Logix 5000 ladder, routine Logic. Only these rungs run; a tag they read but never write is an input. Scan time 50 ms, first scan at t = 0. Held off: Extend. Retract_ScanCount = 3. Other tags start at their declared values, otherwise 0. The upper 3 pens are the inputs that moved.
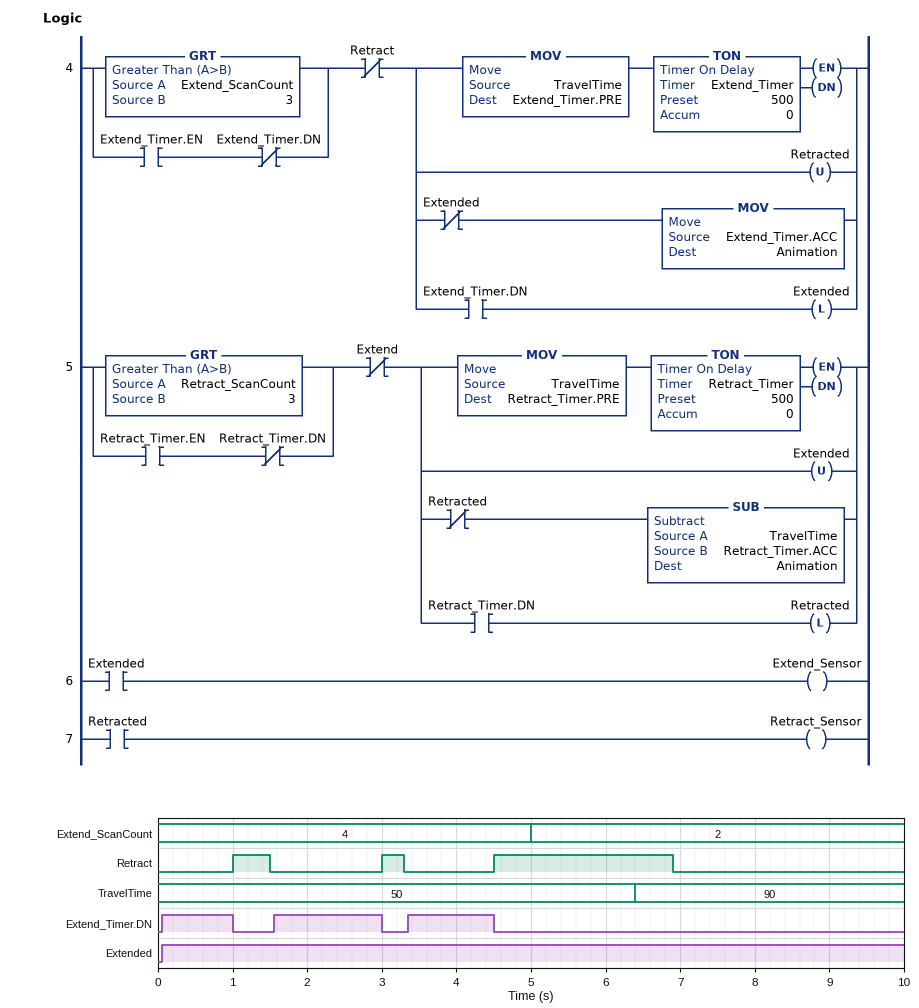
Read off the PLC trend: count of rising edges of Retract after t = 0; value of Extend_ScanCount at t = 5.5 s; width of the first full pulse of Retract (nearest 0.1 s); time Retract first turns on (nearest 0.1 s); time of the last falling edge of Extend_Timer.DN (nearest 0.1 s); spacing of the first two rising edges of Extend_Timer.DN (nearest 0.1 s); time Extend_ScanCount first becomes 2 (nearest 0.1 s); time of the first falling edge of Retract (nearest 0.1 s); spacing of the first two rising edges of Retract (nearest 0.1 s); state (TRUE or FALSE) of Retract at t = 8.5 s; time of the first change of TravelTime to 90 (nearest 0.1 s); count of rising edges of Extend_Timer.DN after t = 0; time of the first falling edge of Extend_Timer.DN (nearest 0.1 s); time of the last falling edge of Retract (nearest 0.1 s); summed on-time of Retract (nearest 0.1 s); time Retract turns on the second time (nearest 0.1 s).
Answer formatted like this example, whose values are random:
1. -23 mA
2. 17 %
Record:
1. 3
2. 2
3. 0.5 s
4. 1.0 s
5. 4.5 s
6. 1.5 s
7. 5.0 s
8. 1.5 s
9. 2.0 s
10. FALSE
11. 6.4 s
12. 3
13. 1.0 s
14. 6.9 s
15. 3.2 s
16. 3.0 s
